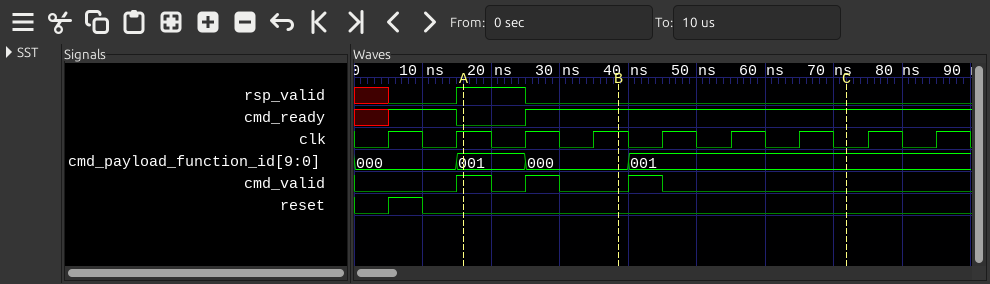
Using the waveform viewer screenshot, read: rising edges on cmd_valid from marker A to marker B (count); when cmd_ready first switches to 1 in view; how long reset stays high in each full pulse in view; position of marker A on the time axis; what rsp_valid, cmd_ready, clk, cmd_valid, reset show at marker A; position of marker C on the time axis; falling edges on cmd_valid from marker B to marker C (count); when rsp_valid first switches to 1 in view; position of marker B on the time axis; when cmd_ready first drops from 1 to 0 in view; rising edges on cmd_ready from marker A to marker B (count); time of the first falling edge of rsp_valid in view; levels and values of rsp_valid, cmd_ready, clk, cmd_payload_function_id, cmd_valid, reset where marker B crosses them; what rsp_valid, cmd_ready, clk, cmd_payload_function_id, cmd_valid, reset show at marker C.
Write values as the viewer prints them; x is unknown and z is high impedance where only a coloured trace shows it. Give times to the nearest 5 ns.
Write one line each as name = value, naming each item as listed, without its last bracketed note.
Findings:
rising edges on cmd_valid from marker A to marker B = 1
when cmd_ready first switches to 1 in view = 5 ns
how long reset stays high in each full pulse in view = 5 ns
position of marker A on the time axis = 15 ns
what rsp_valid, cmd_ready, clk, cmd_valid, reset show at marker A = rsp_valid=1, cmd_ready=0, clk=1, cmd_valid=1, reset=0
position of marker C on the time axis = 70 ns
falling edges on cmd_valid from marker B to marker C = 1
when rsp_valid first switches to 1 in view = 15 ns
position of marker B on the time axis = 40 ns
when cmd_ready first drops from 1 to 0 in view = 15 ns
rising edges on cmd_ready from marker A to marker B = 1
time of the first falling edge of rsp_valid in view = 25 ns
levels and values of rsp_valid, cmd_ready, clk, cmd_payload_function_id, cmd_valid, reset where marker B crosses them = rsp_valid=0, cmd_ready=1, clk=1, cmd_payload_function_id=000, cmd_valid=0, reset=0
what rsp_valid, cmd_ready, clk, cmd_payload_function_id, cmd_valid, reset show at marker C = rsp_valid=0, cmd_ready=1, clk=0, cmd_payload_function_id=001, cmd_valid=0, reset=0
